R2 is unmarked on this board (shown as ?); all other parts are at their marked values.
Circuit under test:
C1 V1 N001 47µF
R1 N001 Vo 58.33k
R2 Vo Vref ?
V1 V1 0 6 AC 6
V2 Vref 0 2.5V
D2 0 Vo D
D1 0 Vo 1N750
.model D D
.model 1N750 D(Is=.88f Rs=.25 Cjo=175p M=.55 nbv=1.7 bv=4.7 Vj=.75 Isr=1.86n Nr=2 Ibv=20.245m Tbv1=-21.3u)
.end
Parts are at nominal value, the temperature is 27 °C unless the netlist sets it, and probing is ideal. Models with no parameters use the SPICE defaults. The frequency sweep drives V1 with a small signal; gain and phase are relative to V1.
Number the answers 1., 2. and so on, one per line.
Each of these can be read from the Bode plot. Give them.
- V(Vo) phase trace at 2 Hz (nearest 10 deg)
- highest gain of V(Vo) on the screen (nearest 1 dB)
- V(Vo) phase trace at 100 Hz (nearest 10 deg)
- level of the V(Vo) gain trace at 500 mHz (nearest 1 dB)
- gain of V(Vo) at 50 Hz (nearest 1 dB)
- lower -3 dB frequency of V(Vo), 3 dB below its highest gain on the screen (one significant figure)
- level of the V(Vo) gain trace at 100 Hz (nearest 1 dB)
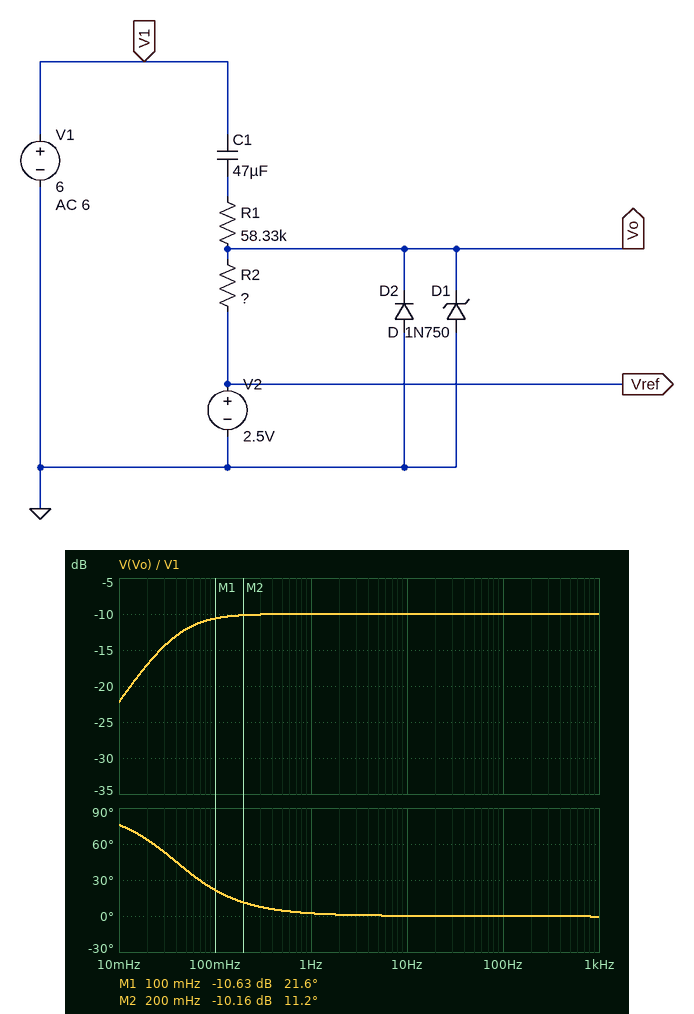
1. 0 deg
2. -10 dB
3. 0 deg
4. -10 dB
5. -10 dB
6. 40 mHz
7. -10 dB
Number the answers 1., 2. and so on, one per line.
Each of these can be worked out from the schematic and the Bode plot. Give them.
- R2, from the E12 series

1. 27 kΩ
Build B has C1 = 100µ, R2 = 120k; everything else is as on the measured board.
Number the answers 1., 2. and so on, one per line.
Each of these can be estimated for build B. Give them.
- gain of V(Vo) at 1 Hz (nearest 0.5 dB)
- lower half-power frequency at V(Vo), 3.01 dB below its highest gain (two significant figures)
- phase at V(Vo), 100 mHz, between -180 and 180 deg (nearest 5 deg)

1. -3.5 dB
2. 8.9 mHz
3. 5 deg
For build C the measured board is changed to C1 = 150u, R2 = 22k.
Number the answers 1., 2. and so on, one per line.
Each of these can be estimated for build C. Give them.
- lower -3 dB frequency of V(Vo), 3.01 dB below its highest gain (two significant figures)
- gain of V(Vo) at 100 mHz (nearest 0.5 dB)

1. 13 mHz
2. -11.5 dB
